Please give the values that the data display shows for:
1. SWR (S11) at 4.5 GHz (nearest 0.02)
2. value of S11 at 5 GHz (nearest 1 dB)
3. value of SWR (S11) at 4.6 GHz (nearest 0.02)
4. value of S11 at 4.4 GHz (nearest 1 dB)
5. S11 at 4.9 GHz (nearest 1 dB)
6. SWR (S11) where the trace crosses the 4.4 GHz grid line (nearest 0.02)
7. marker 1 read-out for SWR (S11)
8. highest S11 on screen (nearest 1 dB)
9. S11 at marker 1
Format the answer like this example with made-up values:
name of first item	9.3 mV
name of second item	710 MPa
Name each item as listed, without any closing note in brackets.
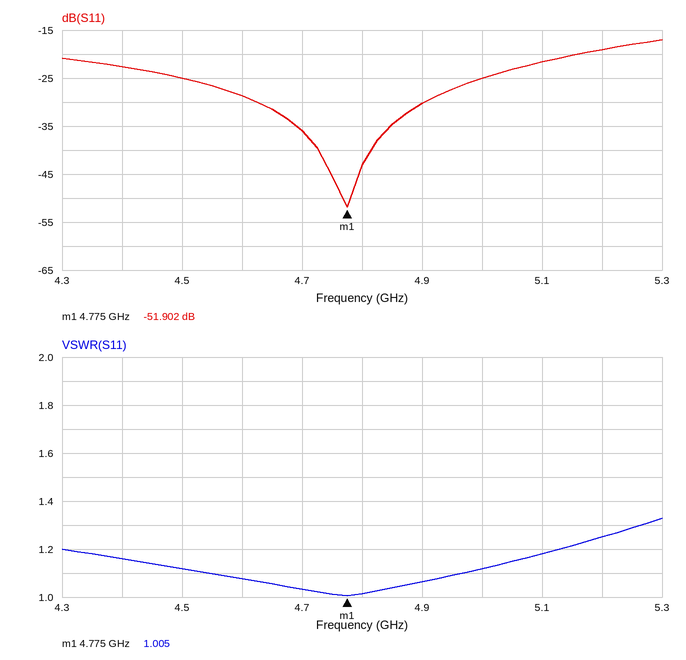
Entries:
SWR (S11) at 4.5 GHz	1.12
value of S11 at 5 GHz	-25 dB
value of SWR (S11) at 4.6 GHz	1.08
value of S11 at 4.4 GHz	-23 dB
S11 at 4.9 GHz	-30 dB
SWR (S11) where the trace crosses the 4.4 GHz grid line	1.16
marker 1 read-out for SWR	1.005
highest S11 on screen	-17 dB
S11 at marker 1	-51.902 dB
